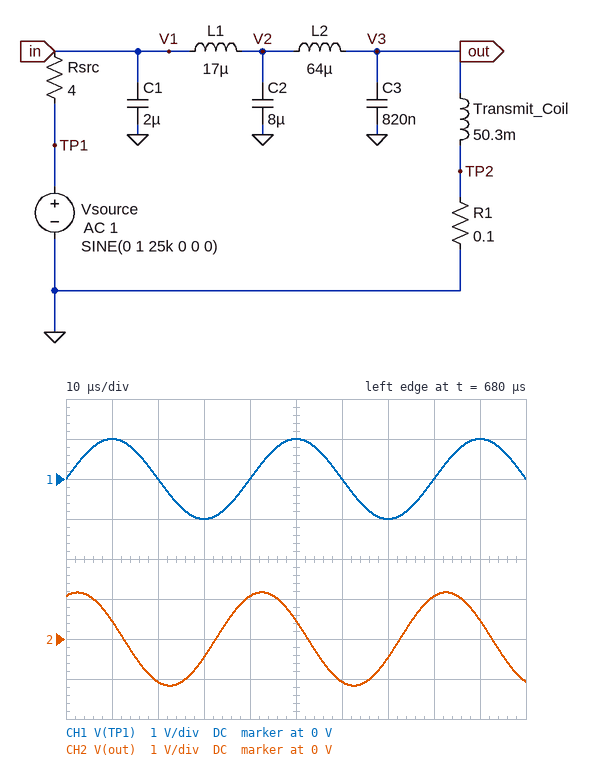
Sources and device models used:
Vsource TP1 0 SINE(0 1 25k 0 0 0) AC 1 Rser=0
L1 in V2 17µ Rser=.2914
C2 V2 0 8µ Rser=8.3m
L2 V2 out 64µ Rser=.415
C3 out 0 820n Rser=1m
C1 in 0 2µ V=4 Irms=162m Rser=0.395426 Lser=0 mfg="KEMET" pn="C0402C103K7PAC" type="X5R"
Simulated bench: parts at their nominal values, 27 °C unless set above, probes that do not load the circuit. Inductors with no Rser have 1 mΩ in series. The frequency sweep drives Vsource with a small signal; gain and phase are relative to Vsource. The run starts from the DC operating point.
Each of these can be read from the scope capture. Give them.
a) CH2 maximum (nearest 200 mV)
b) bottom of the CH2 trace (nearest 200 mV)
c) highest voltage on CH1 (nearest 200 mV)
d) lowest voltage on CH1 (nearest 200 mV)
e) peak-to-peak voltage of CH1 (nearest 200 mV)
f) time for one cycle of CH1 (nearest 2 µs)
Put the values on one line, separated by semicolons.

1.2 V; -1.2 V; 1.0 V; -1.0 V; 2.0 V; 40 µs
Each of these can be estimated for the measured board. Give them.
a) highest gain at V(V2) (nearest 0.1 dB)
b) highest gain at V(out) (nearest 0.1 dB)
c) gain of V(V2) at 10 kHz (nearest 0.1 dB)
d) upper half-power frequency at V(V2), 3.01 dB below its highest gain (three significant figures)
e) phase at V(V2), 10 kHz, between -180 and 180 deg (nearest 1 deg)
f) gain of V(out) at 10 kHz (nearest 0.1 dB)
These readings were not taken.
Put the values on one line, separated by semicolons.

0 dB; 9.0 dB; -8.5 dB; 3.83 kHz; -83 deg; -6.5 dB
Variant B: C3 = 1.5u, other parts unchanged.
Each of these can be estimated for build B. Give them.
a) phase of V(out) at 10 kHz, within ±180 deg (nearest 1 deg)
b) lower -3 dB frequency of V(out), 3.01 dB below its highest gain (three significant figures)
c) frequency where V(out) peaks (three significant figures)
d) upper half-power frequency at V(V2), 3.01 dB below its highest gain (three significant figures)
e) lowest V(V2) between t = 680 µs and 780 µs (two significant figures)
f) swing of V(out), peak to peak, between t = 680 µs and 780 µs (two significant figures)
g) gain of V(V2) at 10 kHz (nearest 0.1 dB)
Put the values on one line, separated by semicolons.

-89 deg; 16.2 kHz; 17.4 kHz; 3.56 kHz; -280 mV; 420 mV; -9.5 dB
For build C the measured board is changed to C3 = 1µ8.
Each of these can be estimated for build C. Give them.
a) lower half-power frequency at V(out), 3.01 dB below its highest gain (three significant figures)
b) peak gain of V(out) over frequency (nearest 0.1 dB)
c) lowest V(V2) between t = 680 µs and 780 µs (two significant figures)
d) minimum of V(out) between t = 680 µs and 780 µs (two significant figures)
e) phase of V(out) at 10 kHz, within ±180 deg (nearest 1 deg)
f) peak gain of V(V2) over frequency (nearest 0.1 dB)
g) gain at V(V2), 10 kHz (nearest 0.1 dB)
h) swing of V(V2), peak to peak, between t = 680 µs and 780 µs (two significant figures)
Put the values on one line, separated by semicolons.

14.8 kHz; 5.7 dB; -280 mV; -150 mV; -91 deg; 0 dB; -10.1 dB; 560 mV
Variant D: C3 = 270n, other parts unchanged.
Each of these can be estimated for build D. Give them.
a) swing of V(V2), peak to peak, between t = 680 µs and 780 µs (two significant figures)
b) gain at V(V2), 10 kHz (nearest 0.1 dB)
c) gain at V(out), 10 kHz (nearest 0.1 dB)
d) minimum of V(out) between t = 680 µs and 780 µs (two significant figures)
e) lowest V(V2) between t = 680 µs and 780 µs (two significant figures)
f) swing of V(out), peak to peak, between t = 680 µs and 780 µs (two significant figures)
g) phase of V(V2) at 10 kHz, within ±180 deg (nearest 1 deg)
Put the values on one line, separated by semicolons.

460 mV; -7.9 dB; -7.3 dB; -410 mV; -230 mV; 810 mV; -81 deg
